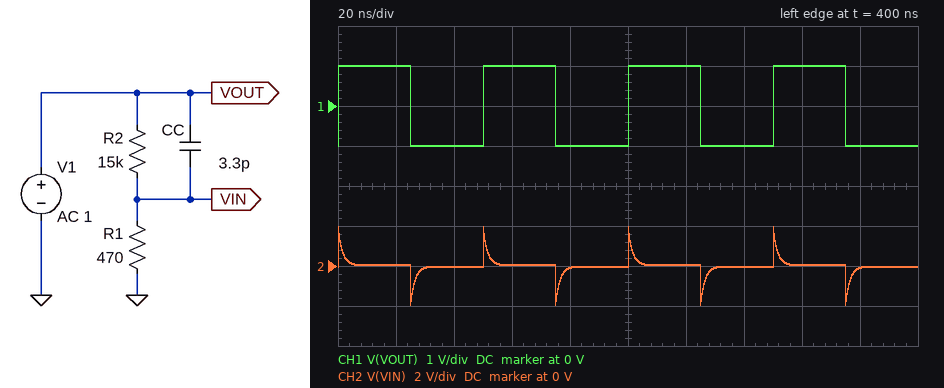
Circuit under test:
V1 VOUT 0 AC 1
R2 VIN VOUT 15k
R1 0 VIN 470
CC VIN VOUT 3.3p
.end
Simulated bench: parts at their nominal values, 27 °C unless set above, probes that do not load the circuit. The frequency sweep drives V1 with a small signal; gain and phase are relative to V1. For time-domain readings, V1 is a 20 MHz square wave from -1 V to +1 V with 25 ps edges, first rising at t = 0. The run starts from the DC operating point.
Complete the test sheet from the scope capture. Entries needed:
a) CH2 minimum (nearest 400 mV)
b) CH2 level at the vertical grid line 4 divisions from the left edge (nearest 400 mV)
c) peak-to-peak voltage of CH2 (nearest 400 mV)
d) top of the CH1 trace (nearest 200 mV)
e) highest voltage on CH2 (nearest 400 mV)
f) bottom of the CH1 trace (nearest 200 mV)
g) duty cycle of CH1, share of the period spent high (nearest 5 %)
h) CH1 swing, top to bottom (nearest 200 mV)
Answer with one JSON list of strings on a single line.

["-2.0 V", "0 V", "4.0 V", "1.0 V", "2.0 V", "-1.0 V", "50 %", "2.0 V"]
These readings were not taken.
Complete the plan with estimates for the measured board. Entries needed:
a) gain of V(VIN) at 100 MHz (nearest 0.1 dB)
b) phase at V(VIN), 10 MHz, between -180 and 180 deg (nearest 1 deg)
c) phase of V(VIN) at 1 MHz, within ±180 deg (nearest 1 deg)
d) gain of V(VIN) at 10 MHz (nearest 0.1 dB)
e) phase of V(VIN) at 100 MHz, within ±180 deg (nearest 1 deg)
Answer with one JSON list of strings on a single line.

["-3.3 dB", "67 deg", "17 deg", "-20.1 dB", "45 deg"]
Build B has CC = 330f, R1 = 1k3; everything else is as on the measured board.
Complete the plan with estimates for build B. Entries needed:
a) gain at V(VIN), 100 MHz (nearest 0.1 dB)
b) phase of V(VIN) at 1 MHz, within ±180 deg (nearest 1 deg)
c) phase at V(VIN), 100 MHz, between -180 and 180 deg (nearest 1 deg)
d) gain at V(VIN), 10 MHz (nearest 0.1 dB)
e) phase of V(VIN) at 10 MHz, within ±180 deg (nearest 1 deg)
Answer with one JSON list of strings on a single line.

["-11.9 dB", "2 deg", "58 deg", "-21.6 dB", "16 deg"]
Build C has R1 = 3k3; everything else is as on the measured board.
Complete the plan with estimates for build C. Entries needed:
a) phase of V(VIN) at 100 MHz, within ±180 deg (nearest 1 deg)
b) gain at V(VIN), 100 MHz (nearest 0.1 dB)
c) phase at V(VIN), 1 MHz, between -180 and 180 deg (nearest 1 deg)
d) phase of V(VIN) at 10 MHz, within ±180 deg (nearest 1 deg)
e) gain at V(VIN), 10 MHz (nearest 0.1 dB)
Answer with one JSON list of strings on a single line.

["8 deg", "-0.1 dB", "14 deg", "43 deg", "-5.8 dB"]
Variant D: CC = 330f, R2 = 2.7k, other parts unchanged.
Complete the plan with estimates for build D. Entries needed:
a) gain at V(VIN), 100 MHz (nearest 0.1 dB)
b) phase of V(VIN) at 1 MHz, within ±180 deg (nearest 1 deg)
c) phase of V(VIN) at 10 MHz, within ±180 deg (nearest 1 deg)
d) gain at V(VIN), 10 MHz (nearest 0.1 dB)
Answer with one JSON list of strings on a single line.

["-15.4 dB", "0 deg", "3 deg", "-16.6 dB"]
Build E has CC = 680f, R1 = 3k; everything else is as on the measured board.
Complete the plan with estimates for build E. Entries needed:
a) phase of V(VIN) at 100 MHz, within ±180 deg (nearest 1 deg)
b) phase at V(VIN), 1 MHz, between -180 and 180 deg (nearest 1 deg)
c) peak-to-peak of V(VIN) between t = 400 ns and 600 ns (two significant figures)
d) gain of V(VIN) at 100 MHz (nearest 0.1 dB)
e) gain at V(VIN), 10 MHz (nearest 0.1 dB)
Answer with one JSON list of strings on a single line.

["34 deg", "3 deg", "3.6 V", "-2.6 dB", "-14.1 dB"]
